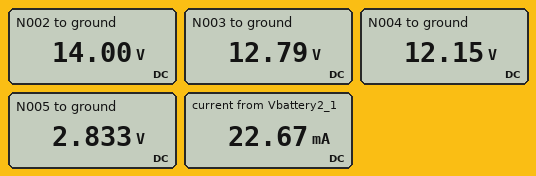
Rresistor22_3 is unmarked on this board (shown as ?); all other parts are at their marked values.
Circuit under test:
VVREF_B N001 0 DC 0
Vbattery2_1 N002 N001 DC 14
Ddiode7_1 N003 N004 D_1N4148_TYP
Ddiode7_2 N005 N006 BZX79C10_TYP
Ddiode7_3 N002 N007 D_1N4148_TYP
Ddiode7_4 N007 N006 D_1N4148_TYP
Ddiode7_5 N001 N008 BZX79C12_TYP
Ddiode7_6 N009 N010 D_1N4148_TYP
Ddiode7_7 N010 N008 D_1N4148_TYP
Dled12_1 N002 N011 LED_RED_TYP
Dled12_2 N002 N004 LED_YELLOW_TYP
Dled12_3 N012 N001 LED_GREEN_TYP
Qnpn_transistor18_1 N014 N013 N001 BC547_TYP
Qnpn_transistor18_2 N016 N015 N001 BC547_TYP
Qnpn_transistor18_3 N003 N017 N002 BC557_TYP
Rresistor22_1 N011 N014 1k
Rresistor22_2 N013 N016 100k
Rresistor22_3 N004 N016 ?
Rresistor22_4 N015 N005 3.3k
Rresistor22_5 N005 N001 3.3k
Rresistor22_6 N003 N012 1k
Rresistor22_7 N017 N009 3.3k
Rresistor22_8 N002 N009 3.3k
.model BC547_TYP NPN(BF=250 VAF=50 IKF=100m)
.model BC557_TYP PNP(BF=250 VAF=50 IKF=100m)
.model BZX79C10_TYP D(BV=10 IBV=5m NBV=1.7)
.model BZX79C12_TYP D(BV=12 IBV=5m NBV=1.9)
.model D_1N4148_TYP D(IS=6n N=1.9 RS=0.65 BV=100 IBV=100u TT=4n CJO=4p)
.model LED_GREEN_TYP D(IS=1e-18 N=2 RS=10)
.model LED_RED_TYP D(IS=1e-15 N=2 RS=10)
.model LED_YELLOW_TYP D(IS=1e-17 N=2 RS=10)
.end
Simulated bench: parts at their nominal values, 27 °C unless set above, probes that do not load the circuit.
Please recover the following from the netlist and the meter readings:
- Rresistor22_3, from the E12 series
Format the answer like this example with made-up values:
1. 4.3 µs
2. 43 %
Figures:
1. 1.2 kΩ
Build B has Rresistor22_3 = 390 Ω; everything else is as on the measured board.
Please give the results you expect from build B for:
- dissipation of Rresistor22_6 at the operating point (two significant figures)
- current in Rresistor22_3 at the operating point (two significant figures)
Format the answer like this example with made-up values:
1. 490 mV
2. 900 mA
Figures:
1. 110 mW
2. 30 mA
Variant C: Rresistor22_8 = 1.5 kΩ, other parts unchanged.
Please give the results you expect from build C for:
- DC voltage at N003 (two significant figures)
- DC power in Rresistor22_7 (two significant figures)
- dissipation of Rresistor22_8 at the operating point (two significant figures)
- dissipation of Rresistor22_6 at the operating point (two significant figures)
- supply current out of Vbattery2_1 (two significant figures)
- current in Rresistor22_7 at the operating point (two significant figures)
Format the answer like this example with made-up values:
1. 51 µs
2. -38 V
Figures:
1. 11 V
2. 4.6 µW
3. 610 µW
4. 80 mW
5. 21 mA
6. 37 µA
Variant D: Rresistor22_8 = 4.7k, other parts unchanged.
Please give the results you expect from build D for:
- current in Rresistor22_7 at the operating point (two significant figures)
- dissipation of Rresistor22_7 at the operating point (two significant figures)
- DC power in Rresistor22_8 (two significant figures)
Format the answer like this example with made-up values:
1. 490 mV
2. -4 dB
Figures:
1. 69 µA
2. 16 µW
3. 250 µW
